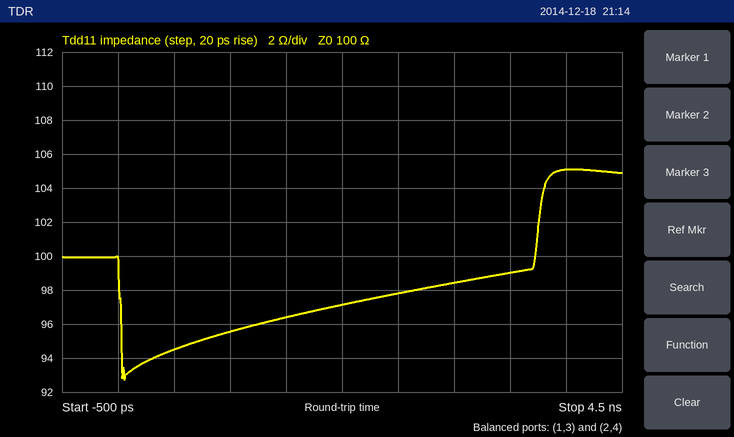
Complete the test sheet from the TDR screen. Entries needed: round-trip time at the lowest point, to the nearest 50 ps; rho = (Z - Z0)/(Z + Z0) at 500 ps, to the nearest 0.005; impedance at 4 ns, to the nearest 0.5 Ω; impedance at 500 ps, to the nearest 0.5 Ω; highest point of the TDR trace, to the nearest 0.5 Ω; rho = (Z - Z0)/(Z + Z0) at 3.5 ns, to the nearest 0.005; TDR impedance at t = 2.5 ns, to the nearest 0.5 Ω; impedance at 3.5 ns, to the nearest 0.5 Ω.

50 ps
-0.030
105.0 Ω
94.5 Ω
105.0 Ω
-0.005
98.0 Ω
99.0 Ω
